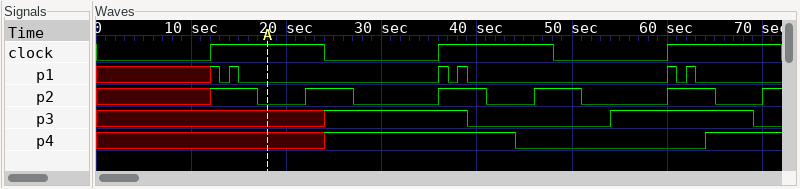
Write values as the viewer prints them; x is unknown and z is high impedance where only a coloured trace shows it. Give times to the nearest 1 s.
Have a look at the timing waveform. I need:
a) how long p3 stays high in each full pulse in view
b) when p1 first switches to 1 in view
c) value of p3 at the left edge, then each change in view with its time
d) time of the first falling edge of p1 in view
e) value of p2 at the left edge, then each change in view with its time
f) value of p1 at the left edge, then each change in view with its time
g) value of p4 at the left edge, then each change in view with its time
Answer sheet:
15 s
12 s
x, 1 at 24 s, 0 at 39 s, 1 at 54 s, 0 at 69 s
13 s
x, 1 at 12 s, 0 at 17 s, 1 at 22 s, 0 at 27 s, 1 at 36 s, 0 at 41 s, 1 at 46 s, 0 at 51 s, 1 at 60 s, 0 at 65 s, 1 at 70 s
x, 1 at 12 s, 0 at 13 s, 1 at 14 s, 0 at 15 s, 1 at 36 s, 0 at 37 s, 1 at 38 s, 0 at 39 s, 1 at 60 s, 0 at 61 s, 1 at 62 s, 0 at 63 s
x, 1 at 24 s, 0 at 44 s, 1 at 64 s
